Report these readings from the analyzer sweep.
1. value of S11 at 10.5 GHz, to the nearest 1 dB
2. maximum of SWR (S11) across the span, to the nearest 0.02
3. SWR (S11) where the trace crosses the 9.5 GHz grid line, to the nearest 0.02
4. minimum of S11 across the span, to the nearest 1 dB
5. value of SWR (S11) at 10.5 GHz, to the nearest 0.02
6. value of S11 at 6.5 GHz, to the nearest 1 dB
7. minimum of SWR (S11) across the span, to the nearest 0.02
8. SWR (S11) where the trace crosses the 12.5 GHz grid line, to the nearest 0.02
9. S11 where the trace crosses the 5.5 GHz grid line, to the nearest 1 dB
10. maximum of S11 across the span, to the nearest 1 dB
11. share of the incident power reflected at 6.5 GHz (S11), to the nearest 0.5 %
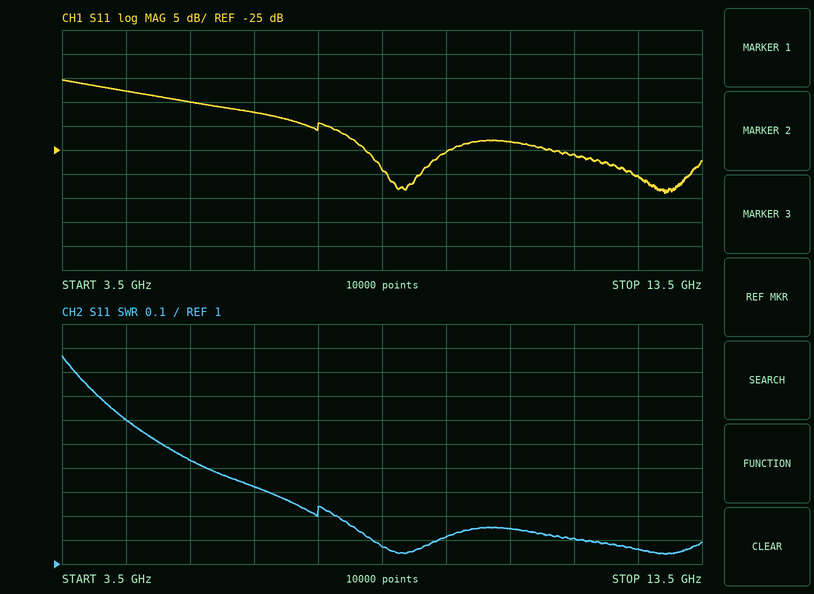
-23 dB
1.86
1.12
-34 dB
1.14
-17 dB
1.04
1.06
-15 dB
-10 dB
2.0 %
